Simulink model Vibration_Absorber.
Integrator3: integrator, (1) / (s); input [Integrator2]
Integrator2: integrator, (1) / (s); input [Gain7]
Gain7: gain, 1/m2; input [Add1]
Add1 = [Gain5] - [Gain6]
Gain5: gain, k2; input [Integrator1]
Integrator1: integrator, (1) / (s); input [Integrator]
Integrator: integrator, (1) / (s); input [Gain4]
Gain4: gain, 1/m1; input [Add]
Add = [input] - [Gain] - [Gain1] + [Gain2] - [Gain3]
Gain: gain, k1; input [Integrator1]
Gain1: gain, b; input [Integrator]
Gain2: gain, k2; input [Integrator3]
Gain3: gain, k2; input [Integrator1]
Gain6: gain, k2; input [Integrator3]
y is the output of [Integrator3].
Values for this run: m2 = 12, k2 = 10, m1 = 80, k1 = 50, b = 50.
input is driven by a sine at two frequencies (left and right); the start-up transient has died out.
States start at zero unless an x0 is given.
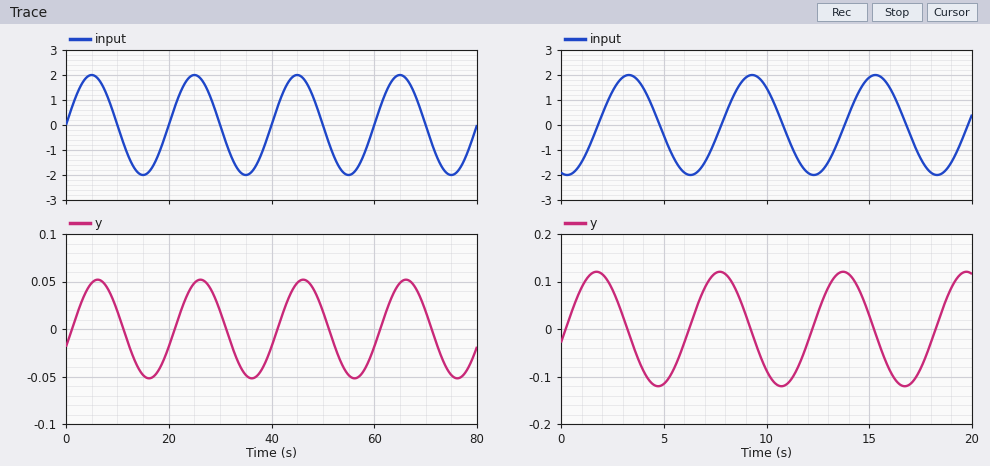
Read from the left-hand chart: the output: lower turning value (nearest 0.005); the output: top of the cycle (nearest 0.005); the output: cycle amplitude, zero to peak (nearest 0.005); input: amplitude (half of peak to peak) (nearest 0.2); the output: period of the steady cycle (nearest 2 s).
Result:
-0.050
0.050
0.050
2.0
20 s
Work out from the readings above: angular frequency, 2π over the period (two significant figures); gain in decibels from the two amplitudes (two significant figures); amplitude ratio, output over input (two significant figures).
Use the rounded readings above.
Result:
0.31 rad/s
-32 dB
0.025
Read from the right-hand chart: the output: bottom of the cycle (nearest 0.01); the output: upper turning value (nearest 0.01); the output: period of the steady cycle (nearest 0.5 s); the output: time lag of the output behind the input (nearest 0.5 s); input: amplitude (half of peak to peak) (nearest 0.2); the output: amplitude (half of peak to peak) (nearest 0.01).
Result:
-0.12
0.12
6.0 s
4.5 s
2.0
0.12
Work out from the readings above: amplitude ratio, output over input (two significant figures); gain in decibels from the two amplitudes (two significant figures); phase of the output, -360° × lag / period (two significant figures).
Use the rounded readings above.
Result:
0.060
-24 dB
-270°
